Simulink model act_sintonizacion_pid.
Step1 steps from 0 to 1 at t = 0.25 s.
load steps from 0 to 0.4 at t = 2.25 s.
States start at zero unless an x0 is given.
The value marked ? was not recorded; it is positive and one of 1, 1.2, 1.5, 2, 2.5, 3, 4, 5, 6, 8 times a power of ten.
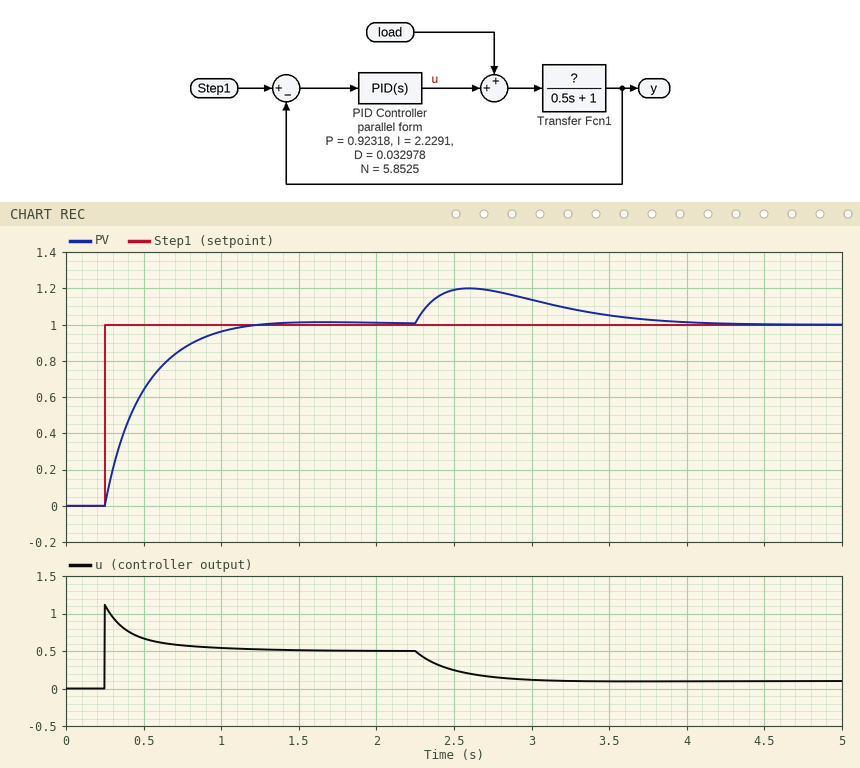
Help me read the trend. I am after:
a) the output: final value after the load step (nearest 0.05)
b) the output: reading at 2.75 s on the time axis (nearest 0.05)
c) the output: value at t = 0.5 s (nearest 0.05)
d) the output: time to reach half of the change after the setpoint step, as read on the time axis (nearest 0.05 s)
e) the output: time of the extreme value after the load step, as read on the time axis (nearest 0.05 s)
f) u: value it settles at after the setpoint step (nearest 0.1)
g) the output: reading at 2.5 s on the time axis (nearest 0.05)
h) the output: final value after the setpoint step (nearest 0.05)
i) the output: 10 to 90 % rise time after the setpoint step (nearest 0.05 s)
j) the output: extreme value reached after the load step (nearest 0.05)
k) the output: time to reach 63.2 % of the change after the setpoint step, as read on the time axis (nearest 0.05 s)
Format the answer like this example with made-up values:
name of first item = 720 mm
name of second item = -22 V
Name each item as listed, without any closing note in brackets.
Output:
the output: final value after the load step = 1.00
the output: reading at 2.75 s on the time axis = 1.20
the output: value at t = 0.5 s = 0.65
the output: time to reach half of the change after the setpoint step, as read on the time axis = 0.40 s
the output: time of the extreme value after the load step, as read on the time axis = 2.60 s
u: value it settles at after the setpoint step = 0.5
the output: reading at 2.5 s on the time axis = 1.20
the output: final value after the setpoint step = 1.00
the output: 10 to 90 % rise time after the setpoint step = 0.55 s
the output: extreme value reached after the load step = 1.20
the output: time to reach 63.2 % of the change after the setpoint step, as read on the time axis = 0.50 s
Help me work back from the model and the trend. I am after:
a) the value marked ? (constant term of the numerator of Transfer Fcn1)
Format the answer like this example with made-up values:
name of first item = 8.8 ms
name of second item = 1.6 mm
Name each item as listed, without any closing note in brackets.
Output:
the value marked ? = 2
